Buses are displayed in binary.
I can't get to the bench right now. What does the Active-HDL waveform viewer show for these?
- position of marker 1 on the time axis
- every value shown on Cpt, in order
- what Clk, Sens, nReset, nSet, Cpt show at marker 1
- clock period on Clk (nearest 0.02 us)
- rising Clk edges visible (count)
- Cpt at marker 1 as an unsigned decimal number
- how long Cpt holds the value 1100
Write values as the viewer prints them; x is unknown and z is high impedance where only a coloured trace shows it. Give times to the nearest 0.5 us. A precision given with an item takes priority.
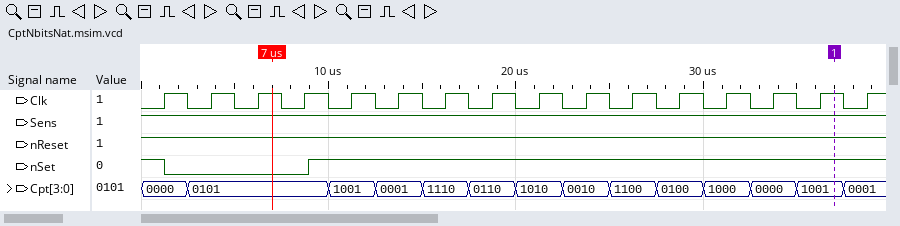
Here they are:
37 us
0000, 0101, 1001, 0001, 1110, 0110, 1010, 0010, 1100, 0100, 1000, 0000, 1001, 0001
Clk=1, Sens=1, nReset=1, nSet=1, Cpt=1001
2.5 us
16
9
2.5 us
